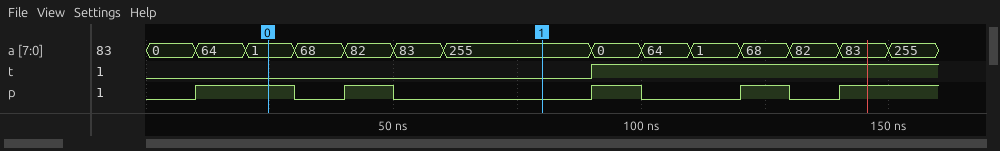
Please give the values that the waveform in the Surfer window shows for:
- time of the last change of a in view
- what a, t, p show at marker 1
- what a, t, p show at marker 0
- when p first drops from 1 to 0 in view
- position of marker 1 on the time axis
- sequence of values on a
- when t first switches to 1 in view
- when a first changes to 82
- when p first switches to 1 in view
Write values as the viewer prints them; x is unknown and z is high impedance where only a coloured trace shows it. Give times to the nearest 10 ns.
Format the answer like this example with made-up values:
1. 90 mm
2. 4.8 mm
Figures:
1. 150 ns
2. a=255, t=0, p=0
3. a=1, t=0, p=1
4. 30 ns
5. 80 ns
6. 0, 64, 1, 68, 82, 83, 255, 0, 64, 1, 68, 82, 83, 255
7. 90 ns
8. 40 ns
9. 10 ns
